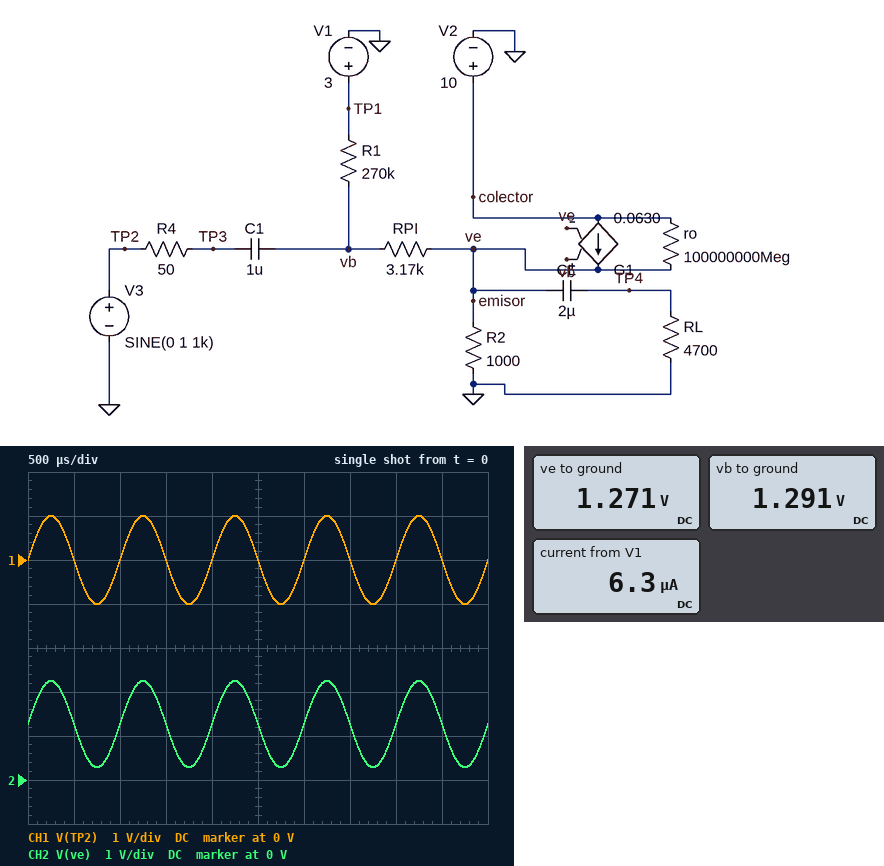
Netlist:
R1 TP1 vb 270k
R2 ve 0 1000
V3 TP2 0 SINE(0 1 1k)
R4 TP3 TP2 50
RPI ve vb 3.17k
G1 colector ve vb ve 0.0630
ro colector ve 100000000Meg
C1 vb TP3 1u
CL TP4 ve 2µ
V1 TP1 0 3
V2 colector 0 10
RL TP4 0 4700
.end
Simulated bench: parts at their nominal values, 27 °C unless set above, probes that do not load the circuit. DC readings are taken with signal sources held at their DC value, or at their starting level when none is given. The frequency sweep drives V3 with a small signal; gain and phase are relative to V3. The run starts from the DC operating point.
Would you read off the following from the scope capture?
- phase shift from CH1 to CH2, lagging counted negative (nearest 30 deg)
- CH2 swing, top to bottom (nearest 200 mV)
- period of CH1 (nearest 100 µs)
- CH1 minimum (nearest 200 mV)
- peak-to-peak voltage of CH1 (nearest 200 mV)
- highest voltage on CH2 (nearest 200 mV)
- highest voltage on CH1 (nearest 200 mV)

0 deg
2.0 V
1.0 ms
-1.0 V
2.0 V
2.2 V
1.0 V
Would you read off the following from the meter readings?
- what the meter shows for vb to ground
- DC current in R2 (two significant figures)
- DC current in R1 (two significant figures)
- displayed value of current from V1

1.291 V
1.3 mA
6.3 µA
6.3 µA
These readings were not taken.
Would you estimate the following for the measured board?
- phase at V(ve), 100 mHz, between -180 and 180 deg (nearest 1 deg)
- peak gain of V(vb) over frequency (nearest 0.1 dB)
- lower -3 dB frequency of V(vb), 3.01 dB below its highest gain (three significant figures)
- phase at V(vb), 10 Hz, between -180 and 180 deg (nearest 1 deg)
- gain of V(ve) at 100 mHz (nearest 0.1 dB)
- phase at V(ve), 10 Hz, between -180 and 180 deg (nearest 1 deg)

86 deg
0 dB
1.38 Hz
8 deg
-22.9 dB
8 deg
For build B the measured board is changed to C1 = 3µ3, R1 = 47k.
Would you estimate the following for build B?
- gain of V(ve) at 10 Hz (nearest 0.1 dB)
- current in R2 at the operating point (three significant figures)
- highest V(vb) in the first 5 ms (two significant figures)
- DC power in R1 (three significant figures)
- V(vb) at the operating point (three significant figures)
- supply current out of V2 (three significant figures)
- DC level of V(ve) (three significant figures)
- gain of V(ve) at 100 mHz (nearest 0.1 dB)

-0.2 dB
2.40 mA
3.4 V
6.72 µW
2.44 V
2.39 mA
2.40 V
-22.2 dB
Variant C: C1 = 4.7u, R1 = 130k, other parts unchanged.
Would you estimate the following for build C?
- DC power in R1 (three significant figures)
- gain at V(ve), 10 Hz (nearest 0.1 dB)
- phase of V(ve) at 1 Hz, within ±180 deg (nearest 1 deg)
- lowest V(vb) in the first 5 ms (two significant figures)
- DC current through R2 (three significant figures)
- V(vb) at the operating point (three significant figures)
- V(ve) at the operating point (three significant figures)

10.5 µW
-0.2 dB
23 deg
830 mV
1.80 mA
1.83 V
1.80 V
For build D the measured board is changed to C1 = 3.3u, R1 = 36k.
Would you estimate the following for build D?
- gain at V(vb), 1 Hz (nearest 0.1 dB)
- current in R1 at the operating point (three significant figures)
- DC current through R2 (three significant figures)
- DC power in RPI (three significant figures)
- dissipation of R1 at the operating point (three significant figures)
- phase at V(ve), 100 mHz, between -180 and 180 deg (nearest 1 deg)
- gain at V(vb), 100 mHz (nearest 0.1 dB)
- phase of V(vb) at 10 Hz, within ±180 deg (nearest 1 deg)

-5.4 dB
12.5 µA
2.51 mA
496 nW
5.63 µW
86 deg
-24.0 dB
9 deg
